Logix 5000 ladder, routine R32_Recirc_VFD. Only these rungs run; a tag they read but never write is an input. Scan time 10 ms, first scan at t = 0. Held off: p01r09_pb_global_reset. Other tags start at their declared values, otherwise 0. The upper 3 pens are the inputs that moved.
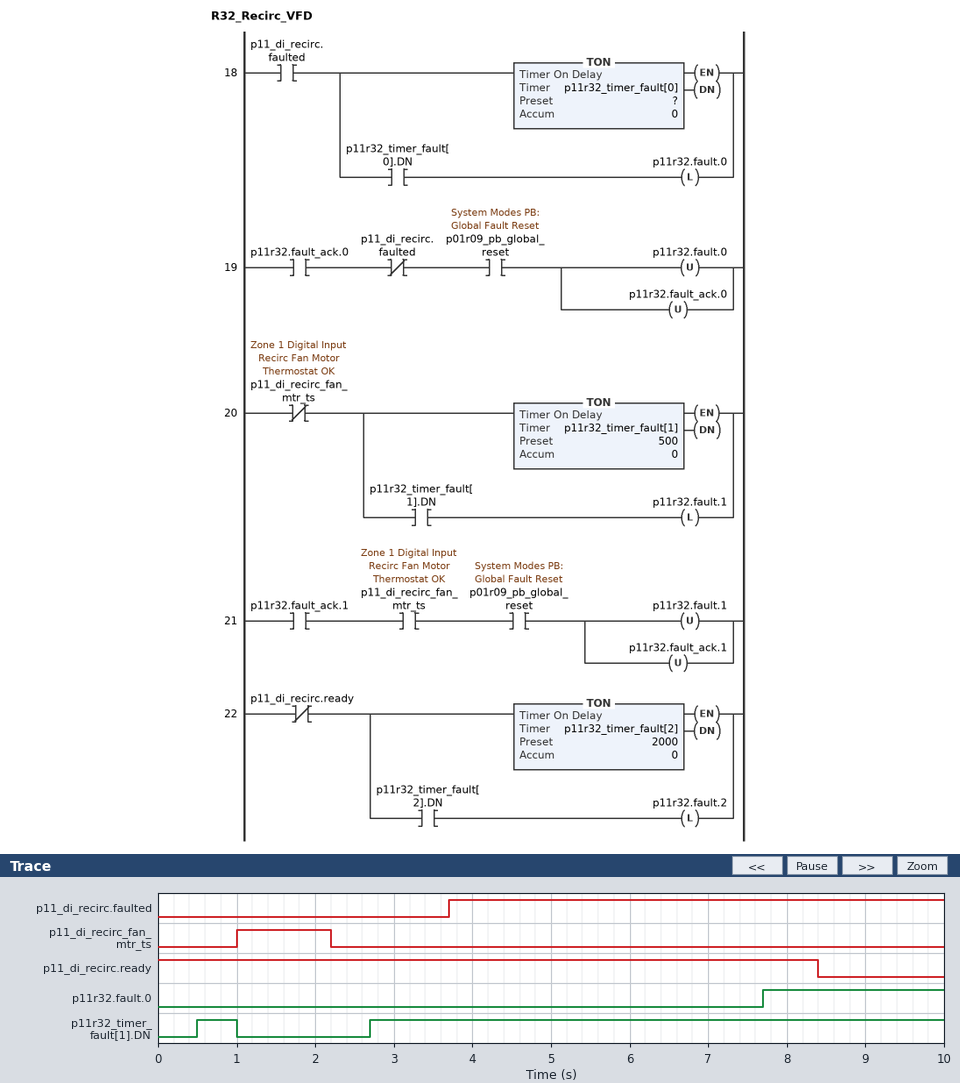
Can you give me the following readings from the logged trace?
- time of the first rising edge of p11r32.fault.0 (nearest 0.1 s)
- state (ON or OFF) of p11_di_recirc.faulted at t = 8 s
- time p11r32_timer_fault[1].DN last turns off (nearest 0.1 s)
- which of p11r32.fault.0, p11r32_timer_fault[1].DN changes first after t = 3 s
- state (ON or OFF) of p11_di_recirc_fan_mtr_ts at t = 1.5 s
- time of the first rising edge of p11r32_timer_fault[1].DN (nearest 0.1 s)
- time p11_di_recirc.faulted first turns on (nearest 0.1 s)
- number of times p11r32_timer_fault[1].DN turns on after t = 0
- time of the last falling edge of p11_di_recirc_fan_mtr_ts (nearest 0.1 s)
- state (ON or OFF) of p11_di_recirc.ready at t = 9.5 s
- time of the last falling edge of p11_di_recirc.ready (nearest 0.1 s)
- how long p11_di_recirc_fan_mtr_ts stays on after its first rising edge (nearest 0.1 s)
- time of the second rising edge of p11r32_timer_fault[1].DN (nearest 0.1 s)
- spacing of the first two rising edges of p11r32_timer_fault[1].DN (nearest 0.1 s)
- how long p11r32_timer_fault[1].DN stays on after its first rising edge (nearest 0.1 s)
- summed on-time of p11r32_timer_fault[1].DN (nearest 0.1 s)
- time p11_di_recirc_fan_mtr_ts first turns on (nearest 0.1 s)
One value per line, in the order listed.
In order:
7.7 s
ON
1.0 s
p11r32.fault.0
ON
0.5 s
3.7 s
2
2.2 s
OFF
8.4 s
1.2 s
2.7 s
2.2 s
0.5 s
7.8 s
1.0 s
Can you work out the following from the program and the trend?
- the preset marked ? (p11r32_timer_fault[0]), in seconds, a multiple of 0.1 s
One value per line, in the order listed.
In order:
4.0 s
